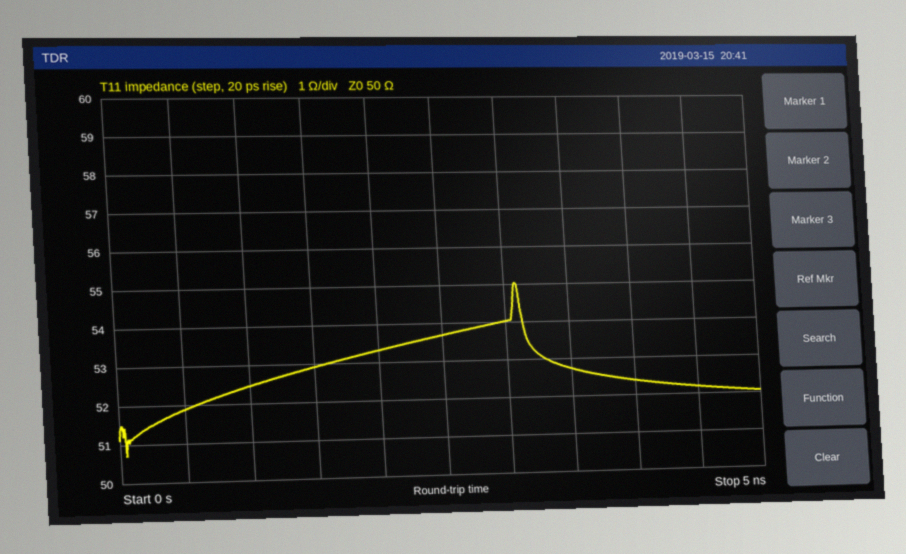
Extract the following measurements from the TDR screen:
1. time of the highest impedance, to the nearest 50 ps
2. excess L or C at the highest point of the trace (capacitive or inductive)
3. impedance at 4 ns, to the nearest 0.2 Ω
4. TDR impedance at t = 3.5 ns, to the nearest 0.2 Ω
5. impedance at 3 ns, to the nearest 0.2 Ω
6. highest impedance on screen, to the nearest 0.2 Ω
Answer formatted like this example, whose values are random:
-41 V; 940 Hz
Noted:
3.10 ns; inductive; 52.4 Ω; 52.8 Ω; 54.0 Ω; 55.0 Ω
